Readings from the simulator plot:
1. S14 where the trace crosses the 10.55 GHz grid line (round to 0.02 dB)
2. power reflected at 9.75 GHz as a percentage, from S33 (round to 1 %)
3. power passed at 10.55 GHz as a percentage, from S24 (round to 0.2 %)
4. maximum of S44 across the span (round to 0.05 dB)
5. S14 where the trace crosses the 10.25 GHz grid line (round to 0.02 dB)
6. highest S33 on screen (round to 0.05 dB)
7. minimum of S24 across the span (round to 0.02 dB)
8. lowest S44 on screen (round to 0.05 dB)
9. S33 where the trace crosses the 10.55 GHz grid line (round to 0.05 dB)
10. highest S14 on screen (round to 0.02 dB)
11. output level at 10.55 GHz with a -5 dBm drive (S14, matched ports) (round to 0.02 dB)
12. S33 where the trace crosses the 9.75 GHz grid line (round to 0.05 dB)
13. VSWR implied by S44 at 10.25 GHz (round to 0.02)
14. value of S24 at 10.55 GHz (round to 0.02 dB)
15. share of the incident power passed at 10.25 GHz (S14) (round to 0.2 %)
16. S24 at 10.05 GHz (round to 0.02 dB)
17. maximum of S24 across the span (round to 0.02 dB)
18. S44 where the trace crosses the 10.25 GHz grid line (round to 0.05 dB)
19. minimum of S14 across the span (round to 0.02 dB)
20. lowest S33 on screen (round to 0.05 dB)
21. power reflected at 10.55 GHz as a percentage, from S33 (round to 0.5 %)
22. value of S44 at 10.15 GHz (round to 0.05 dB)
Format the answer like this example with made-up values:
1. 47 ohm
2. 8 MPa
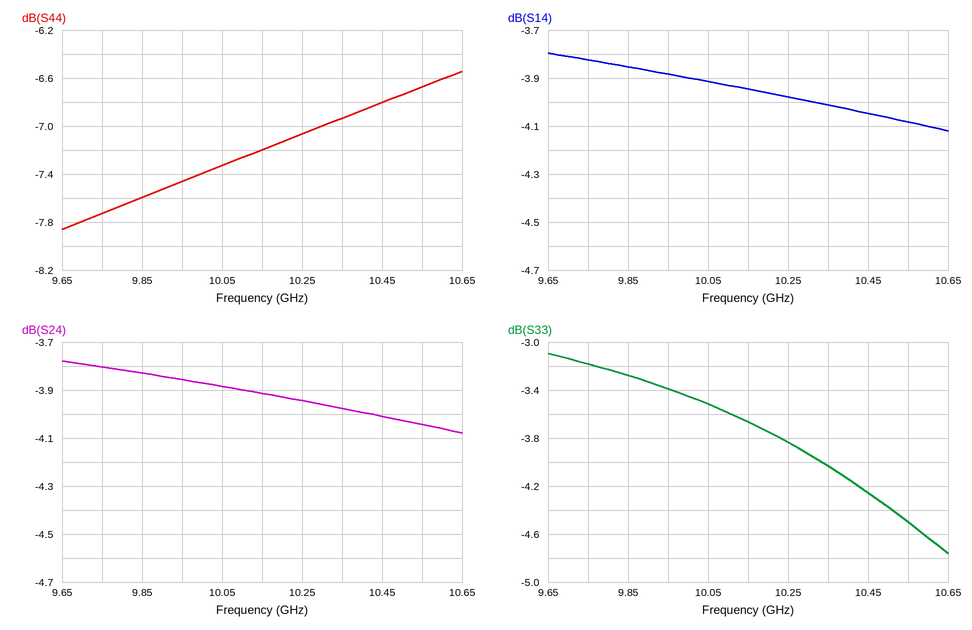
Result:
1. -4.08 dB
2. 48 %
3. 39.4 %
4. -6.55 dB
5. -3.98 dB
6. -3.10 dB
7. -4.08 dB
8. -7.85 dB
9. -4.50 dB
10. -3.80 dB
11. -9.08 dBm
12. -3.20 dB
13. 2.60
14. -4.04 dB
15. 40.0 %
16. -3.88 dB
17. -3.78 dB
18. -7.05 dB
19. -4.12 dB
20. -4.75 dB
21. 35.5 %
22. -7.20 dB
